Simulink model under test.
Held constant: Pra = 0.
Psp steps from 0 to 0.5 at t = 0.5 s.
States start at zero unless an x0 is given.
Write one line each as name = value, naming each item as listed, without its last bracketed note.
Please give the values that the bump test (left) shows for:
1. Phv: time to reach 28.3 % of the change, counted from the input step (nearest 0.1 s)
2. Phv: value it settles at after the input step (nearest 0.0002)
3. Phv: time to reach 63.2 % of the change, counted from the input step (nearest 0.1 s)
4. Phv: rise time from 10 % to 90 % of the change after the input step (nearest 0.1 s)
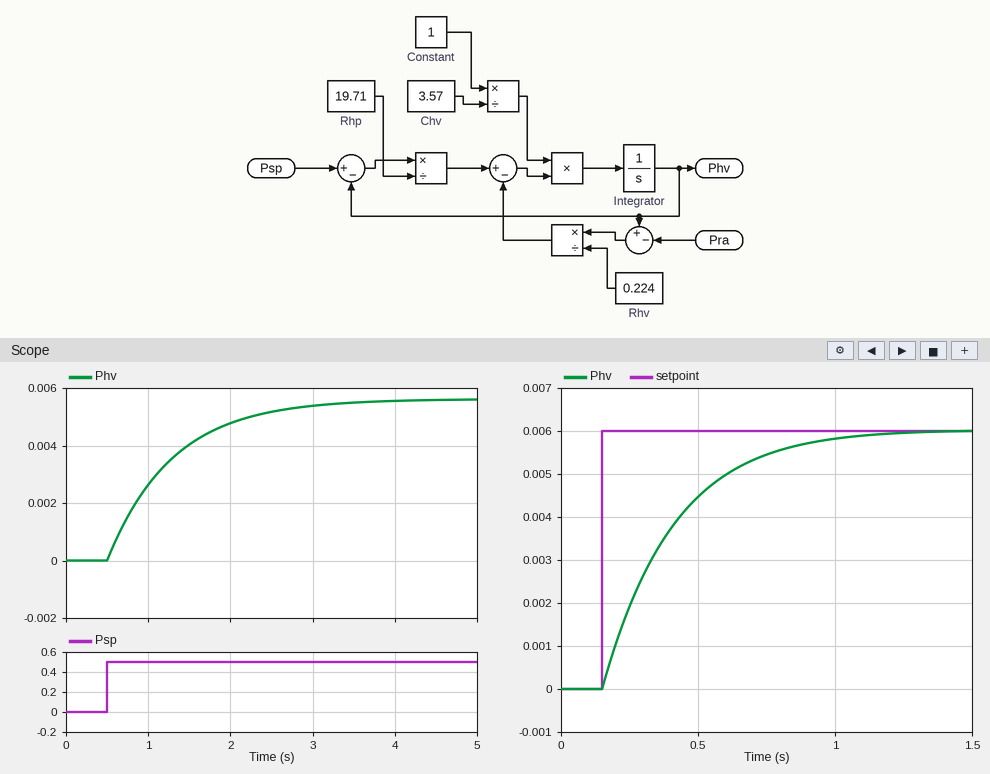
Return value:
Phv: time to reach 28.3 % of the change, counted from the input step = 0.3 s
Phv: value it settles at after the input step = 0.0056
Phv: time to reach 63.2 % of the change, counted from the input step = 0.8 s
Phv: rise time from 10 % to 90 % of the change after the input step = 1.7 s
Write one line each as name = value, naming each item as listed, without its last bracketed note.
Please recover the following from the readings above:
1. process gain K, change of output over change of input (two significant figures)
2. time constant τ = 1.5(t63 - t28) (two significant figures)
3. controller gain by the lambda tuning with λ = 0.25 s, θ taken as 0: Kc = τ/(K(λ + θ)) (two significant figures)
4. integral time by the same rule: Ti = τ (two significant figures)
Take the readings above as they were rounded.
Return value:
process gain K, change of output over change of input = 0.011
time constant τ = 1.5(t63 - t28) = 0.75 s
controller gain by the lambda tuning with λ = 0.25 s, θ taken as 0: Kc = τ/(K(λ + θ)) = 270
integral time by the same rule: Ti = τ = 0.75 s
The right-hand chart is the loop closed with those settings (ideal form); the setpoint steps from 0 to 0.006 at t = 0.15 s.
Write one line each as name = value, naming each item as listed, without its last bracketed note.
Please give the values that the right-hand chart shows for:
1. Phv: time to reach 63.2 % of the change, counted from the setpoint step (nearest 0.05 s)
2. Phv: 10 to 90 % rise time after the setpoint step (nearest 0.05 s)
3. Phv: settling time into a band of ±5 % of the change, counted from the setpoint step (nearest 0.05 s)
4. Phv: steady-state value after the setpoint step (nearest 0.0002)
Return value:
Phv: time to reach 63.2 % of the change, counted from the setpoint step = 0.25 s
Phv: 10 to 90 % rise time after the setpoint step = 0.55 s
Phv: settling time into a band of ±5 % of the change, counted from the setpoint step = 0.75 s
Phv: steady-state value after the setpoint step = 0.0060
